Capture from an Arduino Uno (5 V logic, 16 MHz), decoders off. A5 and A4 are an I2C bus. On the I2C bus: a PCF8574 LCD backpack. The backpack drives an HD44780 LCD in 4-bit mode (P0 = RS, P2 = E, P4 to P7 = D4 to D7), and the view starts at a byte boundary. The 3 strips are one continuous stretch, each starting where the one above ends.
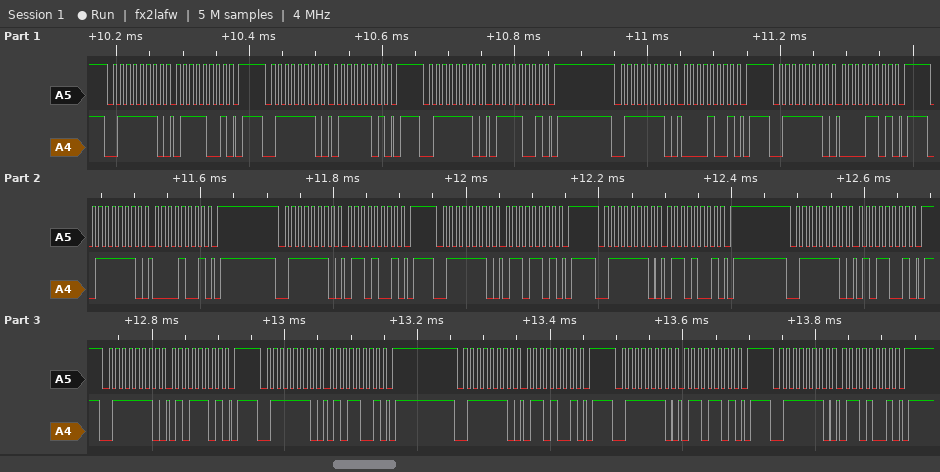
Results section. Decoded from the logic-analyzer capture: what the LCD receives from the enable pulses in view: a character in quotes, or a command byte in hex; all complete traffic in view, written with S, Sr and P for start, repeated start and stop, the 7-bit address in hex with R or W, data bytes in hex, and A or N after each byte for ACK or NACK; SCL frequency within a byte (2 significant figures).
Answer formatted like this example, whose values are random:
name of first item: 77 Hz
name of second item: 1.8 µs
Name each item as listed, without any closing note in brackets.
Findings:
what the LCD receives from the enable pulses in view: a character in quotes, or a command byte in hex: 'p' 'e'
all complete traffic in view, written with S, Sr and P for start, repeated start and stop, the 7-bit address in hex with R or W, data bytes in hex, and A or N after each byte for ACK or NACK: S 3FW A 79 A P S 3FW A 7D A P S 3FW A 79 A P S 3FW A 09 A P S 3FW A 0D A P S 3FW A 09 A P S 3FW A 69 A P S 3FW A 6D A P S 3FW A 69 A P S 3FW A 59 A P S 3FW A 5D A P S 3FW A 59 A P S 3FW A 69 A P S 3FW A 6D A P S 3FW A 69 A P
SCL frequency within a byte: 100 kHz
